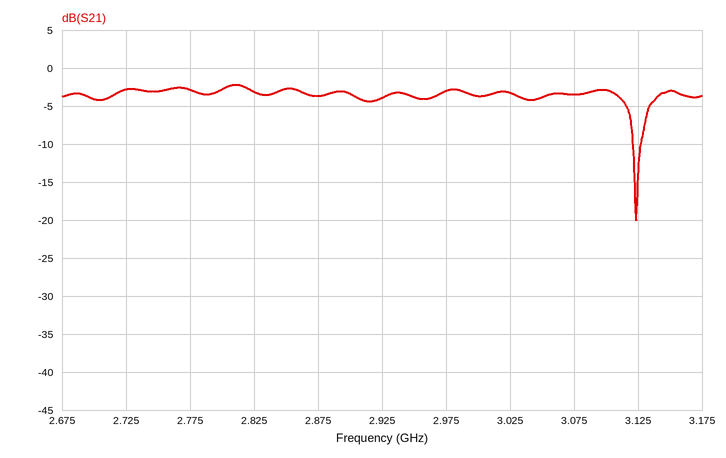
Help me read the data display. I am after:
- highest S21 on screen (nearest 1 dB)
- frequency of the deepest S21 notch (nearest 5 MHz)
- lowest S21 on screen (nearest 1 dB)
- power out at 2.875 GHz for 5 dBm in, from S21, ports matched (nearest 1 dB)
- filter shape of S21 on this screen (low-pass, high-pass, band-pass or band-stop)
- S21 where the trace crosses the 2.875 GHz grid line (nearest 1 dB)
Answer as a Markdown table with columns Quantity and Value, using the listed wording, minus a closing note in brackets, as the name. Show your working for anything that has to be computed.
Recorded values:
| Quantity | Value |
|---|---|
| highest S21 on screen | -2 dB |
| frequency of the deepest S21 notch | 3.125 GHz |
| lowest S21 on screen | -20 dB |
| power out at 2.875 GHz for 5 dBm in, from S21, ports matched | 5 dBm + (-4 dB) = 1 dBm |
| filter shape of S21 on this screen | band-stop |
| S21 where the trace crosses the 2.875 GHz grid line | -4 dB |
